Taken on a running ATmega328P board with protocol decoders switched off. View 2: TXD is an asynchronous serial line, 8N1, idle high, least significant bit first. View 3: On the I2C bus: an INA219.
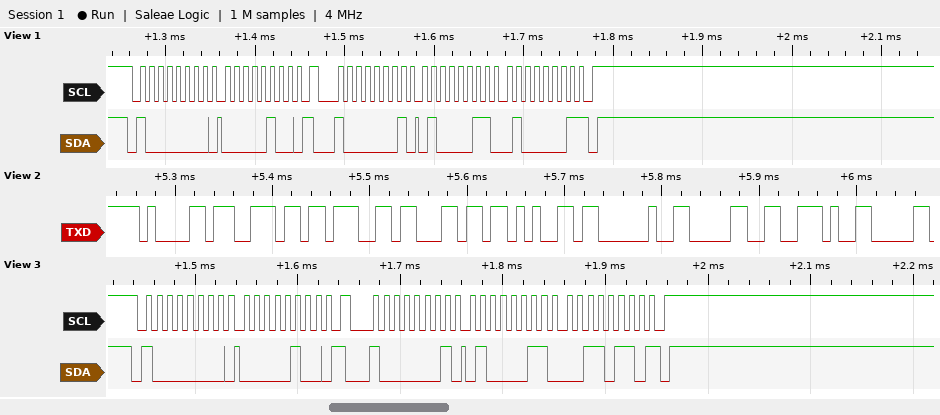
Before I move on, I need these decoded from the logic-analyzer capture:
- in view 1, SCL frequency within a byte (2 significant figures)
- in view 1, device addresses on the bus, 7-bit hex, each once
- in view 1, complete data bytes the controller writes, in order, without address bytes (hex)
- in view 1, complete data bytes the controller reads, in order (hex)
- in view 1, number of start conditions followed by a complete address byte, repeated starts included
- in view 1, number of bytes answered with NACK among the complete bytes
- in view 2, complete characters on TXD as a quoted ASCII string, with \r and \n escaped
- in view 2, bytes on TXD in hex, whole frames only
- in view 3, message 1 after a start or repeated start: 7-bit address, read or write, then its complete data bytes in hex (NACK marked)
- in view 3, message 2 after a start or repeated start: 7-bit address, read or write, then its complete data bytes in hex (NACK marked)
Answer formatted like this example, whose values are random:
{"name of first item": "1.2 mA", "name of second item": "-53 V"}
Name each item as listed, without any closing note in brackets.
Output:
{"in view 1, SCL frequency within a byte": "100 kHz", "in view 1, device addresses on the bus, 7-bit hex, each once": "0x40", "in view 1, complete data bytes the controller writes, in order, without address bytes": "04", "in view 1, complete data bytes the controller reads, in order": "43 41", "in view 1, number of start conditions followed by a complete address byte, repeated starts included": "2", "in view 1, number of bytes answered with NACK among the complete bytes": "1", "in view 2, complete characters on TXD as a quoted ASCII string, with \\r and \\n escaped": "\"angle 0.\"", "in view 2, bytes on TXD in hex, whole frames only": "61 6E 67 6C 65 20 30 2E", "in view 3, message 1 after a start or repeated start: 7-bit address, read or write, then its complete data bytes in hex": "0x40 write: 04", "in view 3, message 2 after a start or repeated start: 7-bit address, read or write, then its complete data bytes in hex": "0x40 read: 43 36 NACK"}
